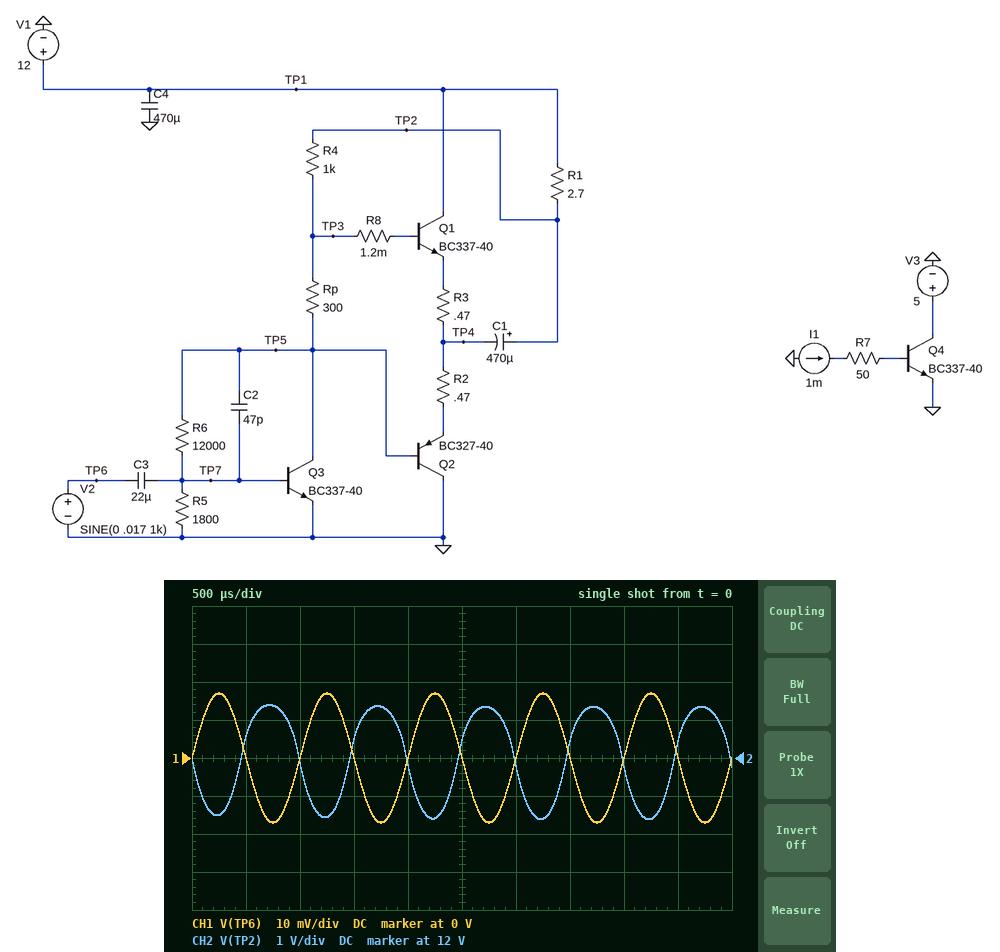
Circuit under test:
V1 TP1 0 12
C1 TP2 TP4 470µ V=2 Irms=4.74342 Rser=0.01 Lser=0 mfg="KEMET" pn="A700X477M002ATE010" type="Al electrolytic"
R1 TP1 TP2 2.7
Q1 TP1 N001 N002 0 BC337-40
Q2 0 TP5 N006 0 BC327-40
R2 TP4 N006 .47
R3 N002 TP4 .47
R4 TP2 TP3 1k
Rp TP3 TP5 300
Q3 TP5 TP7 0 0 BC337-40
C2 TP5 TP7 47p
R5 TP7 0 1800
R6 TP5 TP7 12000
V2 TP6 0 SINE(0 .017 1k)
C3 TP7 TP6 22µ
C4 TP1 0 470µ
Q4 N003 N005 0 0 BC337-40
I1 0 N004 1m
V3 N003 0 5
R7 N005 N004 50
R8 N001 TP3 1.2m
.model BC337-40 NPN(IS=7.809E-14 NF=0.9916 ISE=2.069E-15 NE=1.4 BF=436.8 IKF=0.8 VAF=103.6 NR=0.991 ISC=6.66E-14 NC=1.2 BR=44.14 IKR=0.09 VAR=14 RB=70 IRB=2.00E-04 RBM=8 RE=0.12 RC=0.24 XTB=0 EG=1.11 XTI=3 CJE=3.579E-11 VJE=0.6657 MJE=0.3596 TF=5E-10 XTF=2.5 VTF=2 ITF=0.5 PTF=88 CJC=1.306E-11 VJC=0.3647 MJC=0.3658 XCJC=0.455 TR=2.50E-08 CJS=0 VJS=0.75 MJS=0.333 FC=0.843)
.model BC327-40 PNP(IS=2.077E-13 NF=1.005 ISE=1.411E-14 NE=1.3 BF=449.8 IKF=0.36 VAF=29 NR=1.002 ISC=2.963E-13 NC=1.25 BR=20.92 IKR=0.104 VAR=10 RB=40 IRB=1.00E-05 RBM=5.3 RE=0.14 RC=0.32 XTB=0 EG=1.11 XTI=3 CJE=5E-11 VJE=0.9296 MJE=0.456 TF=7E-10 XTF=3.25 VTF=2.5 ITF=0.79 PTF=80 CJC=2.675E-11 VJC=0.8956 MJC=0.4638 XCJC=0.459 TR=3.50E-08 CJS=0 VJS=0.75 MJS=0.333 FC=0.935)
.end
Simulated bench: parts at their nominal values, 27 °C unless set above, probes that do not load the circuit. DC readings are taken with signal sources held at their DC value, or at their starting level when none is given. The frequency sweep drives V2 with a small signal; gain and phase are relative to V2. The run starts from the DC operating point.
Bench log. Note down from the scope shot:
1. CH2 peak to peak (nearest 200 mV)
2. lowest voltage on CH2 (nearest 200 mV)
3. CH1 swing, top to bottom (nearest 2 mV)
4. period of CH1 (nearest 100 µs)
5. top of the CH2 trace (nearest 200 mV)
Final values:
3.0 V
10.4 V
34 mV
1.0 ms
13.4 V
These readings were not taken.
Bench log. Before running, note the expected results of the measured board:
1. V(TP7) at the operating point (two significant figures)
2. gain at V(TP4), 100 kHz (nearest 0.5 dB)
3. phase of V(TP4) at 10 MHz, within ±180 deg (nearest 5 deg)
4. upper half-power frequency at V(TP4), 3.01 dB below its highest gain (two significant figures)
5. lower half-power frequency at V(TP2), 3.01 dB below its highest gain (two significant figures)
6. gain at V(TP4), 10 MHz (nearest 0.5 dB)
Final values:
640 mV
42.0 dB
55 deg
610 kHz
150 Hz
16.0 dB
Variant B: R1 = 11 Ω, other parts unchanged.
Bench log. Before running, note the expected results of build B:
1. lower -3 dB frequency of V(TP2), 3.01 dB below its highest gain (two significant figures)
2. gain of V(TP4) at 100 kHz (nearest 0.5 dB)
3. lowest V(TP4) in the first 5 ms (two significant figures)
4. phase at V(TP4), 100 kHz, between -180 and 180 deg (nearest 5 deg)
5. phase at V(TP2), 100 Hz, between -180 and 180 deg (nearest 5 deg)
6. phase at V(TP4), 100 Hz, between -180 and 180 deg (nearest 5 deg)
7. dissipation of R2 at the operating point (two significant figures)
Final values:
310 Hz
52.0 dB
1.1 V
165 deg
-90 deg
-110 deg
4.0 mW
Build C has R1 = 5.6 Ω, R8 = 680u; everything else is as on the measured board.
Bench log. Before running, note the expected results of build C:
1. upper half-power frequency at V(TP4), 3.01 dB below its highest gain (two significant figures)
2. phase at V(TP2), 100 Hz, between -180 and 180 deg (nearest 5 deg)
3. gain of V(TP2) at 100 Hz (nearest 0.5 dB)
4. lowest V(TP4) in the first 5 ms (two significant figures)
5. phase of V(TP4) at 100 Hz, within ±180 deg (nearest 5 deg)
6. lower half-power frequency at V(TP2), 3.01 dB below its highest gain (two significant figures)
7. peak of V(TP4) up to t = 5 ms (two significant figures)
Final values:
530 kHz
-90 deg
39.5 dB
2.7 V
-120 deg
220 Hz
8.4 V
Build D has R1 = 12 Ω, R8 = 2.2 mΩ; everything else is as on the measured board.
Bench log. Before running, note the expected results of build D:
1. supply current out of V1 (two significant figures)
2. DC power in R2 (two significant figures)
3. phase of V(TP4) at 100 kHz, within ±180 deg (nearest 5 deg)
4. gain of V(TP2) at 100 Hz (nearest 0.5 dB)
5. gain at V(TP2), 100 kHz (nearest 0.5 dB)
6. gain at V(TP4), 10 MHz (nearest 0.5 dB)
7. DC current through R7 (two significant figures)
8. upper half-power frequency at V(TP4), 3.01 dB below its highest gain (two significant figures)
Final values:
97 mA
3.9 mW
165 deg
41.5 dB
52.5 dB
23.5 dB
1.0 mA
430 kHz
